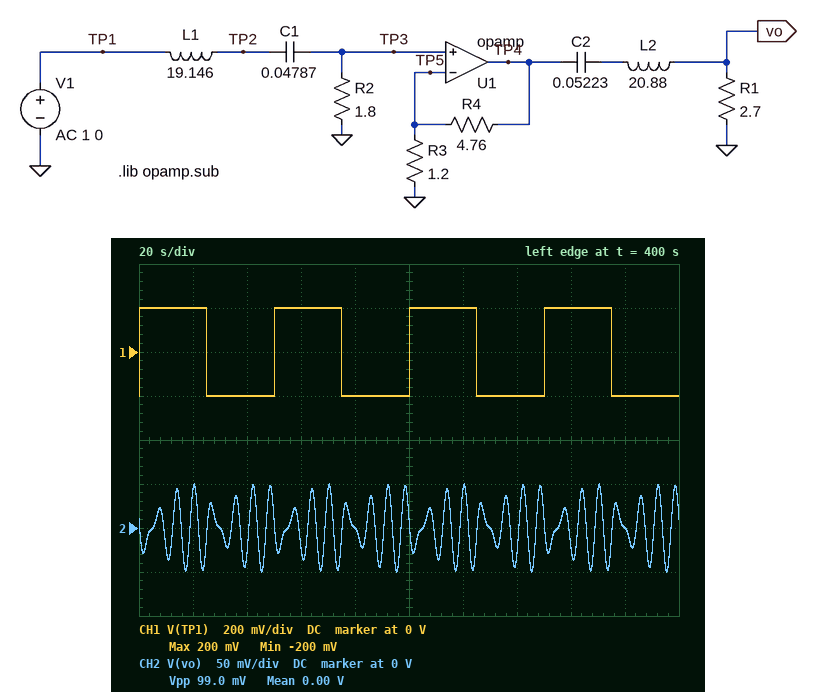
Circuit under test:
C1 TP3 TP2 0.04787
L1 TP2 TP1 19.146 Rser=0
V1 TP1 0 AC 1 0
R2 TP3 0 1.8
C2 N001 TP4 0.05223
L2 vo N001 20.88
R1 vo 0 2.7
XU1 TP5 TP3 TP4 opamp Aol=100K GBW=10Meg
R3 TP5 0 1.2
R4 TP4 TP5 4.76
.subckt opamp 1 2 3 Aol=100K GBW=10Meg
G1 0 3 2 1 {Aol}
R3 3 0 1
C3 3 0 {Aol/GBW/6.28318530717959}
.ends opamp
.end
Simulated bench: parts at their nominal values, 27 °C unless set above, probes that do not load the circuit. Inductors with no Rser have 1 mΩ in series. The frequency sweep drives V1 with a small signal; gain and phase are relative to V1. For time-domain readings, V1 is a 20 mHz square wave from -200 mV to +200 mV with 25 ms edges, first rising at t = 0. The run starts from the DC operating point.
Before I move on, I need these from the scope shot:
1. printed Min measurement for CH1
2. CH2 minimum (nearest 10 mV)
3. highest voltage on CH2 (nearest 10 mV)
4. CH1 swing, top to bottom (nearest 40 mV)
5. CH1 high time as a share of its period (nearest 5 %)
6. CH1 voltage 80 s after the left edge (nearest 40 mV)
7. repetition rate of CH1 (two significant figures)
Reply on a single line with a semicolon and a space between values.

-200 mV; -50 mV; 50 mV; 400 mV; 50 %; -200 mV; 20 mHz
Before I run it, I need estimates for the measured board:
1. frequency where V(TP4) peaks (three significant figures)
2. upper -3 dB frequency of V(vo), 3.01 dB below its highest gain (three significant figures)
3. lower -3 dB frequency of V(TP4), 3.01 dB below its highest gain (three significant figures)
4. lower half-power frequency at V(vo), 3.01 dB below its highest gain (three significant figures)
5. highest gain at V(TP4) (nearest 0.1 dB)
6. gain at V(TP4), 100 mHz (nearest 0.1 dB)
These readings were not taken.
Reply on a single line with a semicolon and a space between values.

166 mHz; 170 mHz; 159 mHz; 152 mHz; 13.9 dB; -7.5 dB
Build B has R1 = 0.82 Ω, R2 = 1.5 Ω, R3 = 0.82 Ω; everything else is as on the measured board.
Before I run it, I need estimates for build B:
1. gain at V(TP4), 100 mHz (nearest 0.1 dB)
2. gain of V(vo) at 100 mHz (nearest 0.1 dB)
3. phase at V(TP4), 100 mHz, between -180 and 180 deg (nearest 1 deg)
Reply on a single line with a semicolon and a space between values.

-6.4 dB; -32.9 dB; 86 deg
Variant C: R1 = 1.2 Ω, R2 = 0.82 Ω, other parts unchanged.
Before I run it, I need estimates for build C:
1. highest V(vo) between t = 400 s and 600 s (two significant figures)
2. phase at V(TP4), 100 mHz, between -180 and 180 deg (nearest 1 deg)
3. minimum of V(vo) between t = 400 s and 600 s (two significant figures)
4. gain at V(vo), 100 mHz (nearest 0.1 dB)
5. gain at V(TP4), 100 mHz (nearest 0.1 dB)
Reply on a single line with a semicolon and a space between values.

14 mV; 88 deg; -14 mV; -37.6 dB; -14.3 dB
